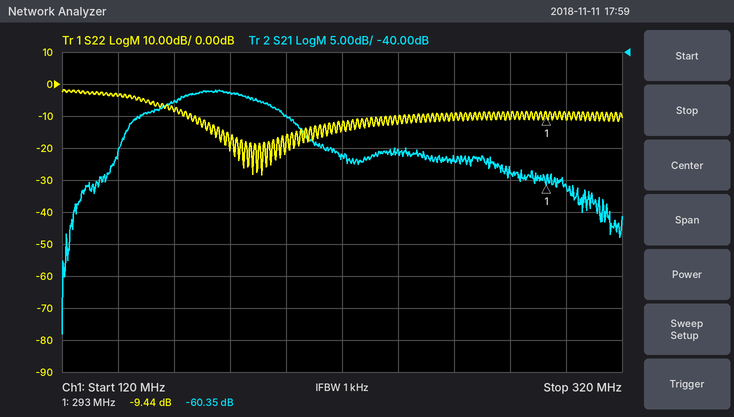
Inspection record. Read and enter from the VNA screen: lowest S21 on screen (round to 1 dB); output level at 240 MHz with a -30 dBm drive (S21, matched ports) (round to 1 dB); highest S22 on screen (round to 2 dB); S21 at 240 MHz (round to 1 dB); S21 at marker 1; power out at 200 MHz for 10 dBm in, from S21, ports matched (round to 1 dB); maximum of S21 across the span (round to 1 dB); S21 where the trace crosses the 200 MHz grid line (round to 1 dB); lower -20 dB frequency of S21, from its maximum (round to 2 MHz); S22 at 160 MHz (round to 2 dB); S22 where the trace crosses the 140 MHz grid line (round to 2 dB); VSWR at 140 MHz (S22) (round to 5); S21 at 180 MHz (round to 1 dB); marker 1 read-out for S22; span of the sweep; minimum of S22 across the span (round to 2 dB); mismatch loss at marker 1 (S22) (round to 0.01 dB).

-84 dB
-85 dBm
-2 dB
-55 dB
-60.35 dB
-40 dBm
-46 dB
-50 dB
124 MHz
-8 dB
-4 dB
5
-46 dB
-9.44 dB
200 MHz
-28 dB
0.52 dB
